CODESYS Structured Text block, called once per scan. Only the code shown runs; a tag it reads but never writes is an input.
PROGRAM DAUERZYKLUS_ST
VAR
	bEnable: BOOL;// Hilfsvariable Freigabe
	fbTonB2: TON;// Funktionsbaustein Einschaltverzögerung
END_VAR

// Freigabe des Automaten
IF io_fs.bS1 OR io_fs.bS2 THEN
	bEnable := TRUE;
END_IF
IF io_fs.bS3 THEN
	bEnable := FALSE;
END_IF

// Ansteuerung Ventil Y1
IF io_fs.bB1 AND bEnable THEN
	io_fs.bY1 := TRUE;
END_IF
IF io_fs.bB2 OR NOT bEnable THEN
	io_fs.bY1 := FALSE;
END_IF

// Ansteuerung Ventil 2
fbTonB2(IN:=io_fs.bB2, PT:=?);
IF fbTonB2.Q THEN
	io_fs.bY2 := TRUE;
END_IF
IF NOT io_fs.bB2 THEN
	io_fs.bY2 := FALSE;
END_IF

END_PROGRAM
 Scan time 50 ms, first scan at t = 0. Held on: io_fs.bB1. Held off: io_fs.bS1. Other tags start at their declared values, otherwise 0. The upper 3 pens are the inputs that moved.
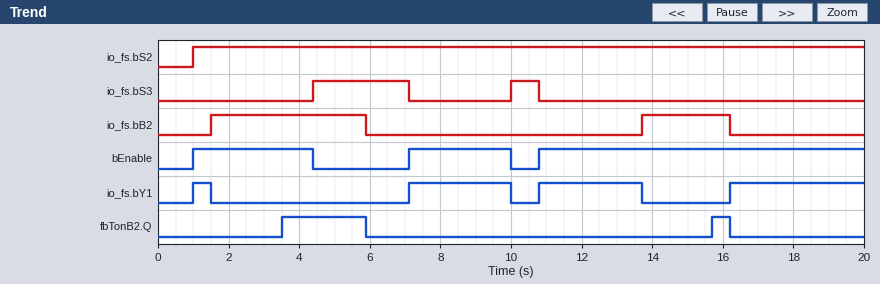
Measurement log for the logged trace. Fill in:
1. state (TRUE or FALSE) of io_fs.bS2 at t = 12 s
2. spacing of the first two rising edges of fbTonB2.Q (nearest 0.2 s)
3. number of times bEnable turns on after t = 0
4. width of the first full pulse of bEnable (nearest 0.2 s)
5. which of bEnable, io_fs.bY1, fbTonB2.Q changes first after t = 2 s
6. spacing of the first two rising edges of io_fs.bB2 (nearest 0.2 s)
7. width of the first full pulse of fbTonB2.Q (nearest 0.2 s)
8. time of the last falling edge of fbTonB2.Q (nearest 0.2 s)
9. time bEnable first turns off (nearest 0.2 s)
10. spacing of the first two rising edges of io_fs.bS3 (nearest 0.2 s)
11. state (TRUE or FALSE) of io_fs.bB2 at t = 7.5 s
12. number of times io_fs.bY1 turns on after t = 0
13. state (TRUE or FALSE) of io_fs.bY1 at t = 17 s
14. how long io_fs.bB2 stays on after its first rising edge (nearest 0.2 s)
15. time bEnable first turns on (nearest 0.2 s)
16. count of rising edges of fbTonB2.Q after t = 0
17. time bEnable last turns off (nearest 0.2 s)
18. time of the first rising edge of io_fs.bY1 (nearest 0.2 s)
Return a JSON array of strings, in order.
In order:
["TRUE", "12.2 s", "3", "3.4 s", "fbTonB2.Q", "12.2 s", "2.4 s", "16.2 s", "4.4 s", "5.6 s", "FALSE", "4", "TRUE", "4.4 s", "1.0 s", "2", "10.0 s", "1.0 s"]
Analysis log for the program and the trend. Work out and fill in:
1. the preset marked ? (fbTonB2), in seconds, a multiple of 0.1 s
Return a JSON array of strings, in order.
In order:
["2.0 s"]
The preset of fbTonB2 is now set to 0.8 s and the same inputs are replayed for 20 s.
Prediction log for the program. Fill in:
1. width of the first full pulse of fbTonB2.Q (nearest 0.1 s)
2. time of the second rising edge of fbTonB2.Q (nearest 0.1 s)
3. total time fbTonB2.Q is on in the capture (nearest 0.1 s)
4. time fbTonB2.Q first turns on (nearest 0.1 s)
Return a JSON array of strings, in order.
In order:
["3.6 s", "14.5 s", "5.3 s", "2.3 s"]
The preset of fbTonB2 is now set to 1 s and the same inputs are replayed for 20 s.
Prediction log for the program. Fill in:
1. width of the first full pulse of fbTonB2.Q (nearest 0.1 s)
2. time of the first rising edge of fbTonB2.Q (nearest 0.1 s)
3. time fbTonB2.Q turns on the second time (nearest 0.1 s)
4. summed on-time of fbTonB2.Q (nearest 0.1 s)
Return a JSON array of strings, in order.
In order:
["3.4 s", "2.5 s", "14.7 s", "4.9 s"]
